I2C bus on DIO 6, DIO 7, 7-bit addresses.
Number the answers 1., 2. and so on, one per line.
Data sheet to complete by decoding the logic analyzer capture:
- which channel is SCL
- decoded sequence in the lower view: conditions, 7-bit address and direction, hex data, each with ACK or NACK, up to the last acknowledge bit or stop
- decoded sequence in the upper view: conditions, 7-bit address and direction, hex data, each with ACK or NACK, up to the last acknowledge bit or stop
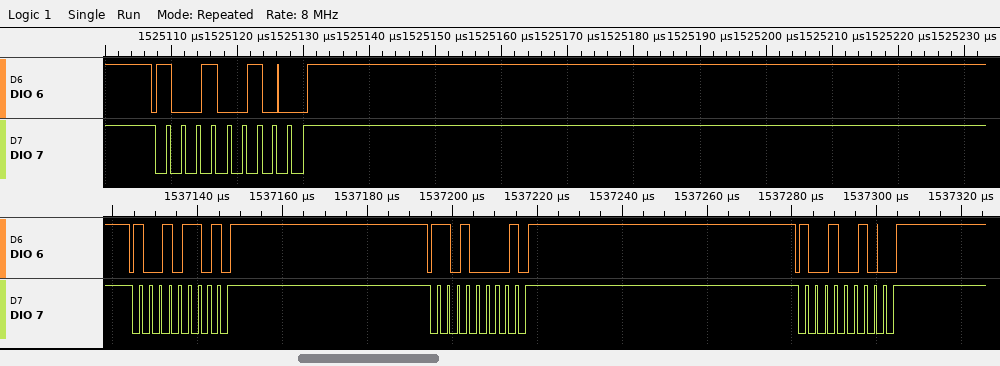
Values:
1. DIO 7
2. start, address 4B write NACK, stop, start, address 68 write NACK, stop, start, address 49 write ACK, stop
3. start, address 49 write ACK, stop
